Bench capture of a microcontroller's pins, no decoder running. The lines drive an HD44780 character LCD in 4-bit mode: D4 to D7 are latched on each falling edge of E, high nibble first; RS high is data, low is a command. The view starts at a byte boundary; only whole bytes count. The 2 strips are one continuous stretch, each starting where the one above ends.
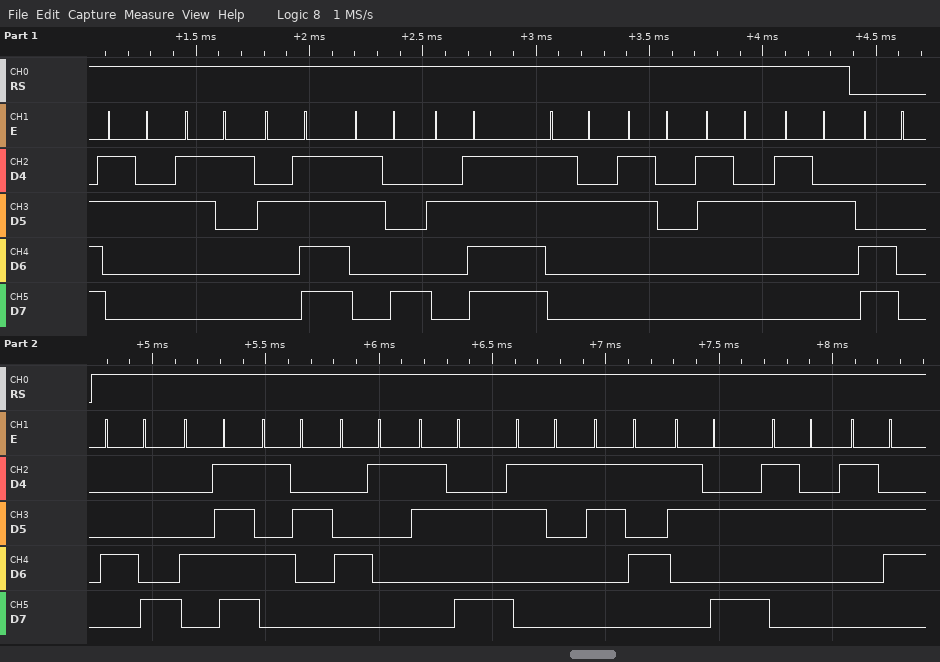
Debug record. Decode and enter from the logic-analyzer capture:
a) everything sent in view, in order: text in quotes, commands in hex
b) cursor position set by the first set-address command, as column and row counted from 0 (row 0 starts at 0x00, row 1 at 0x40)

"21/8/2022" 0xC0 "HORA:15:26"
column 0, row 1
